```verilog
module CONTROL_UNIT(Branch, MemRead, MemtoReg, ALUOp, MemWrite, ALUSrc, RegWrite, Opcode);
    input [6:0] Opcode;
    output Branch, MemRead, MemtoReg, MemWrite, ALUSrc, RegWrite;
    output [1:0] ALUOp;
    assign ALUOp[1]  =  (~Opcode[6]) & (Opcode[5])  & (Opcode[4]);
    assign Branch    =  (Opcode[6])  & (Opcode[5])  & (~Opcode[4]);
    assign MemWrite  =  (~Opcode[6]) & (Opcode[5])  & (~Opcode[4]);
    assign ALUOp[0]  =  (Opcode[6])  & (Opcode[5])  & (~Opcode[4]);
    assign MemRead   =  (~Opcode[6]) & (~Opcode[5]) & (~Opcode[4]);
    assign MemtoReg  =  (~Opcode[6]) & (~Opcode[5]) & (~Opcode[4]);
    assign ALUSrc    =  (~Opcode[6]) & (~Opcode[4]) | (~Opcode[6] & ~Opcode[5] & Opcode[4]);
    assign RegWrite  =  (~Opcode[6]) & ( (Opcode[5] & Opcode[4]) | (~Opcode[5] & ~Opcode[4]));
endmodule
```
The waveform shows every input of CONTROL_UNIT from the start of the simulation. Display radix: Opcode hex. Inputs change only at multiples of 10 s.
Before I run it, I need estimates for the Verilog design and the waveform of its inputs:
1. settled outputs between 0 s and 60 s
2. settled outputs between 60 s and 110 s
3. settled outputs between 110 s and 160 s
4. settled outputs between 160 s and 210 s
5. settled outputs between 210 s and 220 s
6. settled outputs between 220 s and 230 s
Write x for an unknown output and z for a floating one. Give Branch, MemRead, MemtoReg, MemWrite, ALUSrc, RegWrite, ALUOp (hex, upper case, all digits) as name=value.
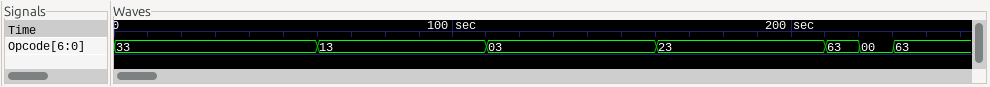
Branch=0, MemRead=0, MemtoReg=0, MemWrite=0, ALUSrc=0, RegWrite=1, ALUOp=2
Branch=0, MemRead=0, MemtoReg=0, MemWrite=0, ALUSrc=1, RegWrite=0, ALUOp=0
Branch=0, MemRead=1, MemtoReg=1, MemWrite=0, ALUSrc=1, RegWrite=1, ALUOp=0
Branch=0, MemRead=0, MemtoReg=0, MemWrite=1, ALUSrc=1, RegWrite=0, ALUOp=0
Branch=1, MemRead=0, MemtoReg=0, MemWrite=0, ALUSrc=0, RegWrite=0, ALUOp=1
Branch=0, MemRead=1, MemtoReg=1, MemWrite=0, ALUSrc=1, RegWrite=1, ALUOp=0
